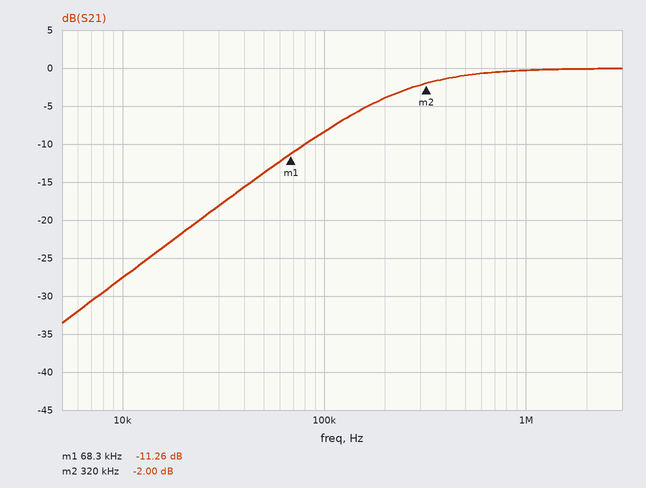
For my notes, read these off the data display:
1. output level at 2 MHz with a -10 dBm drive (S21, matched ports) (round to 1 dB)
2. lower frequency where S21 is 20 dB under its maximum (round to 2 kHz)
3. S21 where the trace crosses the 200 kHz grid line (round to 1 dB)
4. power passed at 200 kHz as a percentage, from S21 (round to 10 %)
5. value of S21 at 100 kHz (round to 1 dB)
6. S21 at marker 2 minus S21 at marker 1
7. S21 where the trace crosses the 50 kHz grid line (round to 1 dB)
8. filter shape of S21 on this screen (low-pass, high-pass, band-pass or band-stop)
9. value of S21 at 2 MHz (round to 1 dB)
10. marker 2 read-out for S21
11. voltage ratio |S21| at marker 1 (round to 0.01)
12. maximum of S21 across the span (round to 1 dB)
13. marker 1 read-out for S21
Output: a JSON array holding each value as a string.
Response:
["-10 dBm", "24 kHz", "-4 dB", "40 %", "-8 dB", "9.26 dB", "-14 dB", "high-pass", "0 dB", "-2.00 dB", "0.27", "0 dB", "-11.26 dB"]
